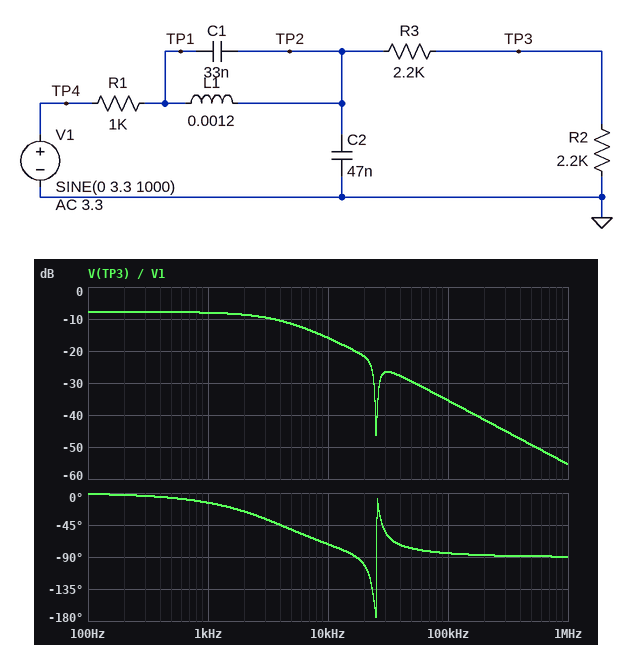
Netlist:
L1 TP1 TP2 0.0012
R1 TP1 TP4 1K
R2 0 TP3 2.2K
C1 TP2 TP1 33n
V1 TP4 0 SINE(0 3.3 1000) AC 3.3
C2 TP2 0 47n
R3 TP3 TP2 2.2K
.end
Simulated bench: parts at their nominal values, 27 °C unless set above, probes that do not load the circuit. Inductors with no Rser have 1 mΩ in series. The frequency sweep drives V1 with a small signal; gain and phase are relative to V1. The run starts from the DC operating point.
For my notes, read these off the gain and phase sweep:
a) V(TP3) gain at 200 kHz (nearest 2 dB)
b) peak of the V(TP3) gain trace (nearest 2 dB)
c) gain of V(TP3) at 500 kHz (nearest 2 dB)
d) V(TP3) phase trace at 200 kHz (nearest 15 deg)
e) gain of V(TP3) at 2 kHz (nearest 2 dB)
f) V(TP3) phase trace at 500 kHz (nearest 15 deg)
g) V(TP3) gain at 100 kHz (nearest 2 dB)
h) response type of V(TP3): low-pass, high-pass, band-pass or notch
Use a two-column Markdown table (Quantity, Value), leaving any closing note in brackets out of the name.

| Quantity | Value |
|---|---|
| V(TP3) gain at 200 kHz | -42 dB |
| peak of the V(TP3) gain trace | -8 dB |
| gain of V(TP3) at 500 kHz | -50 dB |
| V(TP3) phase trace at 200 kHz | -90 deg |
| gain of V(TP3) at 2 kHz | -8 dB |
| V(TP3) phase trace at 500 kHz | -90 deg |
| V(TP3) gain at 100 kHz | -36 dB |
| response type of V(TP3): low-pass, high-pass, band-pass or notch | low-pass |
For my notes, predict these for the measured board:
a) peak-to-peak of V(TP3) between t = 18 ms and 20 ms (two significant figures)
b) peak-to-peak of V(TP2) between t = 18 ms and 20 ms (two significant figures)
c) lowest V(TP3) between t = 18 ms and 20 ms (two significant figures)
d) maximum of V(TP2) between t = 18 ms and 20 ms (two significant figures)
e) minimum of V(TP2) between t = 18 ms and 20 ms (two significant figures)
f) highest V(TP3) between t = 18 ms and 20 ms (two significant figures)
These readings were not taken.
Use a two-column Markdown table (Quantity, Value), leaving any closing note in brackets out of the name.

| Quantity | Value |
|---|---|
| peak-to-peak of V(TP3) between t = 18 ms and 20 ms | 2.6 V |
| peak-to-peak of V(TP2) between t = 18 ms and 20 ms | 5.2 V |
| lowest V(TP3) between t = 18 ms and 20 ms | -1.3 V |
| maximum of V(TP2) between t = 18 ms and 20 ms | 2.6 V |
| minimum of V(TP2) between t = 18 ms and 20 ms | -2.6 V |
| highest V(TP3) between t = 18 ms and 20 ms | 1.3 V |
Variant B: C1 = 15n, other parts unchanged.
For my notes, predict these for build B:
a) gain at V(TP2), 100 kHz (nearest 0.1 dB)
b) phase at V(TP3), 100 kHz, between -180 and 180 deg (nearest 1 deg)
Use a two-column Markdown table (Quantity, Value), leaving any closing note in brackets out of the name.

| Quantity | Value |
|---|---|
| gain at V(TP2), 100 kHz | -29.5 dB |
| phase at V(TP3), 100 kHz, between -180 and 180 deg | -81 deg |
